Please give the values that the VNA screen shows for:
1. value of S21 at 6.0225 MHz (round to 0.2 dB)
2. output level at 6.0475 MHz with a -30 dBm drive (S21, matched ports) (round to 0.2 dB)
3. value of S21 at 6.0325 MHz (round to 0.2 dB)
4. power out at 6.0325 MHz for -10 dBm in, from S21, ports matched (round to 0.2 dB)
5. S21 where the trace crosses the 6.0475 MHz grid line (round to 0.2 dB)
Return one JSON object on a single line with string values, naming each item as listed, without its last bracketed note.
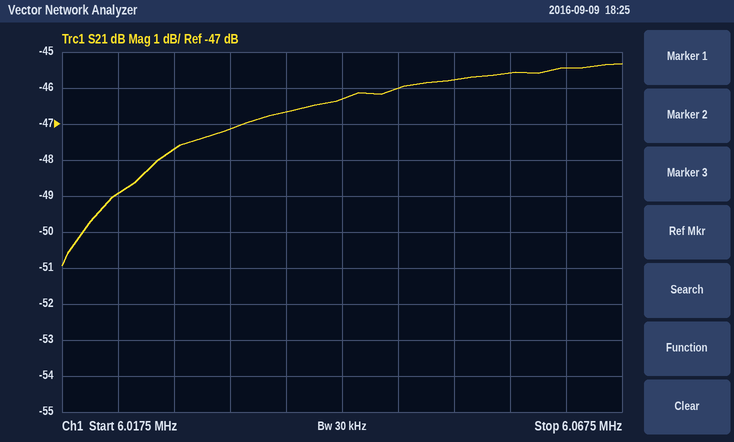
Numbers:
{"value of S21 at 6.0225 MHz": "-49.0 dB", "output level at 6.0475 MHz with a -30 dBm drive (S21, matched ports)": "-76.0 dBm", "value of S21 at 6.0325 MHz": "-47.2 dB", "power out at 6.0325 MHz for -10 dBm in, from S21, ports matched": "-57.2 dBm", "S21 where the trace crosses the 6.0475 MHz grid line": "-46.0 dB"}
